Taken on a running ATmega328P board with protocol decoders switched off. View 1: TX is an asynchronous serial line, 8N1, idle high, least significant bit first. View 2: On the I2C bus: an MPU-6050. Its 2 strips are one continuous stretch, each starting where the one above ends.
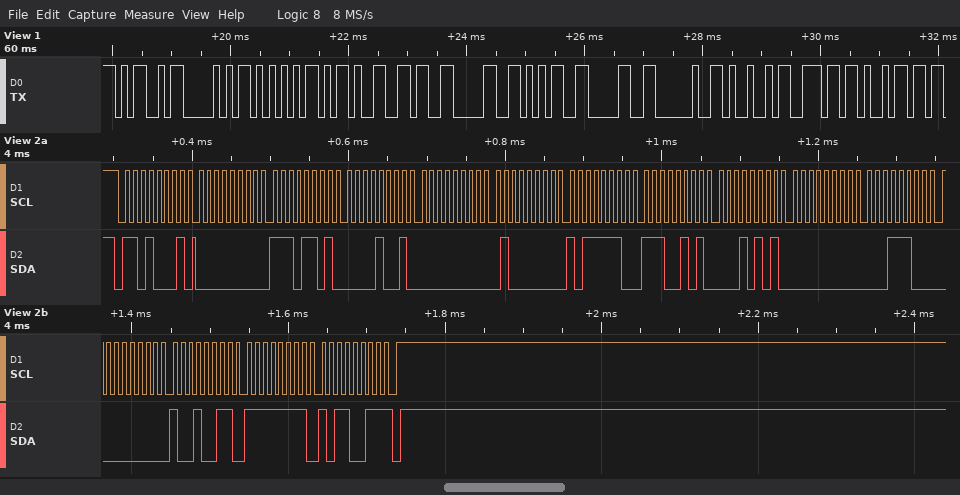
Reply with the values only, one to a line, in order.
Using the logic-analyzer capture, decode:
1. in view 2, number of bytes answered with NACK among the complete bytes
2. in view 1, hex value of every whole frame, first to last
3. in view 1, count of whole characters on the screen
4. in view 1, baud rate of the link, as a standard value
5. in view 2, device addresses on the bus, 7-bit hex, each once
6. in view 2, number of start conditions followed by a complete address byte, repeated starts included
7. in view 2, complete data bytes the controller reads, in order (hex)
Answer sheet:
1
4D 50 55 2D 36 30 35 30 20 49 6E 69
12
9600 baud
0x68
1
00 ED 09 00 40 BE E5 15 00 1C 00 93 FF B3
